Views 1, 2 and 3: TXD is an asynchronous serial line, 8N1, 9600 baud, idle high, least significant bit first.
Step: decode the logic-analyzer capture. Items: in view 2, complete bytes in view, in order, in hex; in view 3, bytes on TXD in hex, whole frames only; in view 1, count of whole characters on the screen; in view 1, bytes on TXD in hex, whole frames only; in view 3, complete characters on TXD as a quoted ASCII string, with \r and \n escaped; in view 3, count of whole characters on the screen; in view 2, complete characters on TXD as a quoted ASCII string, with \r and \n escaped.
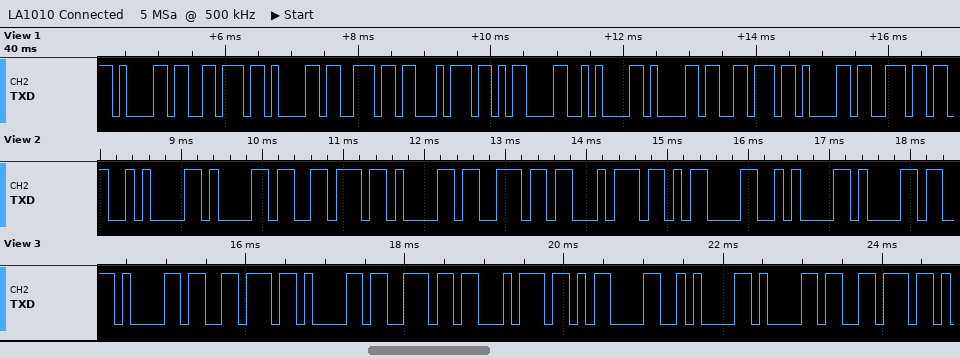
0A 61 76 61 6E 74 0D 0A 61
0x61 0x76 0x61 0x6E 0x74 0x0D 0x0A 0x61 0x76
11
61 76 61 6E 74 0D 0A 61 76 61 6E
"avant\r\nav"
9
"\navant\r\na"
